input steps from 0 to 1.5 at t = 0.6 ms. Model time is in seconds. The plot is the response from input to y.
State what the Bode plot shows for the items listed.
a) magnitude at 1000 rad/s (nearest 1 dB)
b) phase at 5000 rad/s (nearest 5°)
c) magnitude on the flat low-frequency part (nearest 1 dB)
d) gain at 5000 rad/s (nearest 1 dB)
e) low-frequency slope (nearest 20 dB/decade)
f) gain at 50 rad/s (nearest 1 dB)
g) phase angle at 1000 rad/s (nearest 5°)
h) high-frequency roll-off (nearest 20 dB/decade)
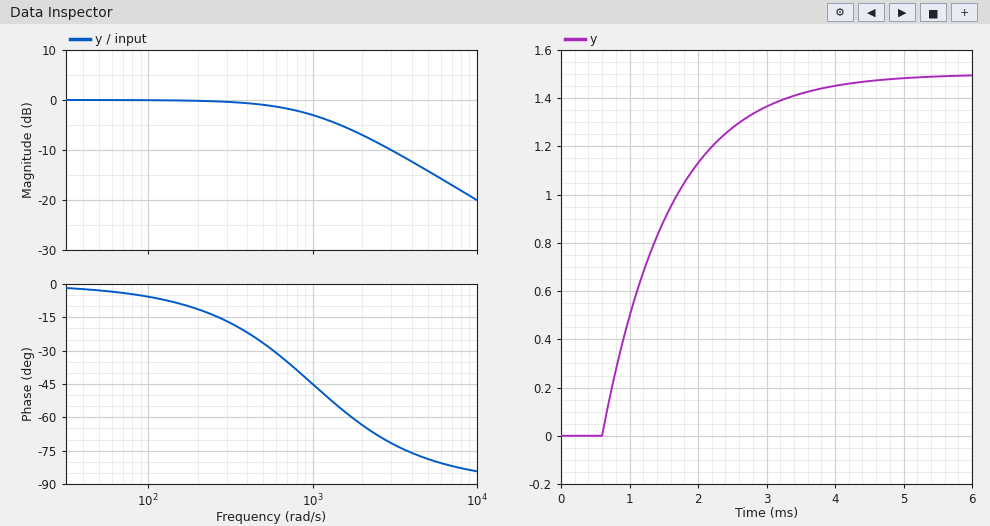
-3 dB
-80°
0 dB
-14 dB
0 dB/decade
0 dB
-45°
-20 dB/decade
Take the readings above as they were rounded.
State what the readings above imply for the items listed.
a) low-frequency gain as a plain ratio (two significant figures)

1.0
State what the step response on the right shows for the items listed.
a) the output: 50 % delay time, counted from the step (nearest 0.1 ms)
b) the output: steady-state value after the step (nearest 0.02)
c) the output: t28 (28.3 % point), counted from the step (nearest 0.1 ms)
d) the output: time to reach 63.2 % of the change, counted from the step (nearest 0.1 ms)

0.7 ms
1.50
0.3 ms
1.0 ms
